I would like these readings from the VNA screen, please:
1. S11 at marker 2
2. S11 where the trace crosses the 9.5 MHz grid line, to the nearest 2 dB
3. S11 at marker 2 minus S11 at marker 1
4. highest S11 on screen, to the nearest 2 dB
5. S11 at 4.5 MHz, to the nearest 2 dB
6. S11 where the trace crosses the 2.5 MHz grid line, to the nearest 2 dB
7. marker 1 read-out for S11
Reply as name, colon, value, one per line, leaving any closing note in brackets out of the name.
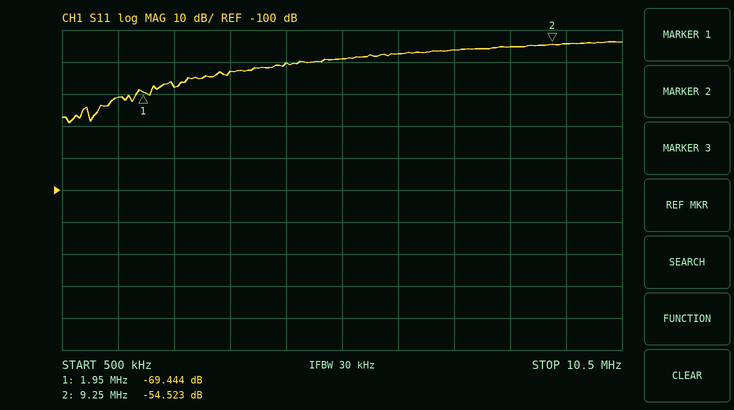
S11 at marker 2: -54.523 dB
S11 where the trace crosses the 9.5 MHz grid line, to the nearest 2 dB: -54 dB
S11 at marker 2 minus S11 at marker 1: 14.921 dB
highest S11 on screen, to the nearest 2 dB: -54 dB
S11 at 4.5 MHz, to the nearest 2 dB: -60 dB
S11 where the trace crosses the 2.5 MHz grid line, to the nearest 2 dB: -68 dB
marker 1 read-out for S11: -69.444 dB
